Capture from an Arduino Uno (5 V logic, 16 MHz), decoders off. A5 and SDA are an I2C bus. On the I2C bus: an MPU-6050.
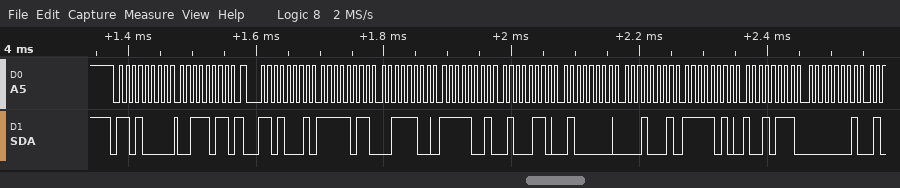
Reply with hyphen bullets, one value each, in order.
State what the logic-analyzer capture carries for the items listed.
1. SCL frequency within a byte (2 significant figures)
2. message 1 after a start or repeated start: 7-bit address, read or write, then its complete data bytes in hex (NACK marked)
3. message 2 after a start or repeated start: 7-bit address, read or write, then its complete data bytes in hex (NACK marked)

- 100 kHz
- 0x68 write: 3B
- 0x68 read: FB 3C F9 46 40 11 FA 97 01
